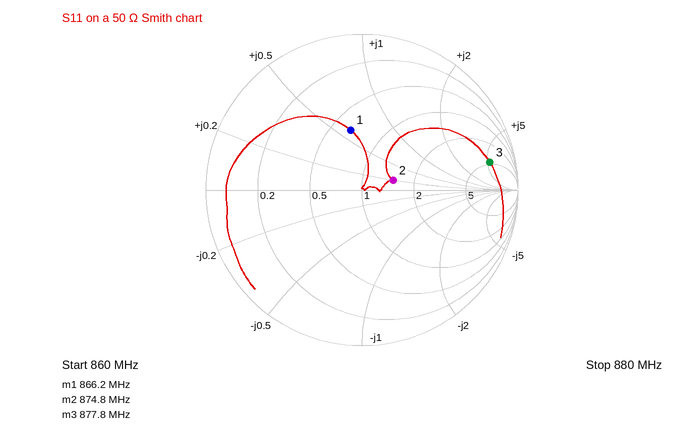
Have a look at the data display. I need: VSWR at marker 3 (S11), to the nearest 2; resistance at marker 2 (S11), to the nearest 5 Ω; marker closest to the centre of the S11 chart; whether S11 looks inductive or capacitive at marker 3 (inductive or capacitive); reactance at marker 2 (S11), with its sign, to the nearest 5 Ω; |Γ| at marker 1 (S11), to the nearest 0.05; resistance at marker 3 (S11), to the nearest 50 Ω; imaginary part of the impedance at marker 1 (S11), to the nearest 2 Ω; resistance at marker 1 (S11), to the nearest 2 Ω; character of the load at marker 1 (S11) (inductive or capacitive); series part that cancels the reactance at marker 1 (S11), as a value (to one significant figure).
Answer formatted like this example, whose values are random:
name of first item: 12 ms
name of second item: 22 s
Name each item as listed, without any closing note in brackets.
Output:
VSWR at marker 3 (S11), to the nearest 2: 12
resistance at marker 2 (S11), to the nearest 5 Ω: 75 Ω
marker closest to the centre of the S11 chart: marker 2
whether S11 looks inductive or capacitive at marker 3: inductive
reactance at marker 2 (S11), with its sign, to the nearest 5 Ω: +10 Ω
|Γ| at marker 1 (S11), to the nearest 0.05: 0.40
resistance at marker 3 (S11), to the nearest 50 Ω: 250 Ω
imaginary part of the impedance at marker 1 (S11), to the nearest 2 Ω: +30 Ω
resistance at marker 1 (S11), to the nearest 2 Ω: 32 Ω
character of the load at marker 1 (S11): inductive
series part that cancels the reactance at marker 1 (S11), as a value: 6 pF
